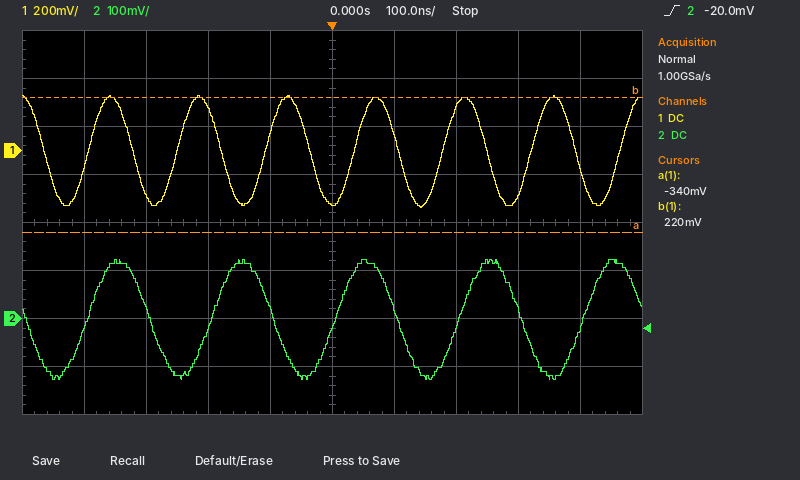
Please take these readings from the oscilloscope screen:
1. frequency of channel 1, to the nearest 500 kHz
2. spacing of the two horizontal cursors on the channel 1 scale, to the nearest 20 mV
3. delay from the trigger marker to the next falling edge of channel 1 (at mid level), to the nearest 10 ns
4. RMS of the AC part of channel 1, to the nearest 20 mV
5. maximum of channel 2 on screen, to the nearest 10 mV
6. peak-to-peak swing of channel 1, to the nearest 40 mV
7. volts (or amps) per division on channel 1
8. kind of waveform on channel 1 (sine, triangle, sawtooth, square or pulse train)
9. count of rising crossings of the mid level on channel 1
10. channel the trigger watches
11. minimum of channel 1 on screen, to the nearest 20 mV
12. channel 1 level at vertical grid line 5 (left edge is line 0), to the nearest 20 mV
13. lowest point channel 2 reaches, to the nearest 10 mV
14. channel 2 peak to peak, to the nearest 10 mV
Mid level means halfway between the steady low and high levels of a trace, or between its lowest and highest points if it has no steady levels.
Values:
7.0 MHz
560 mV
110 ns
160 mV
120 mV
480 mV
200 mV
sine
7
channel 2
-240 mV
-220 mV
-130 mV
250 mV
